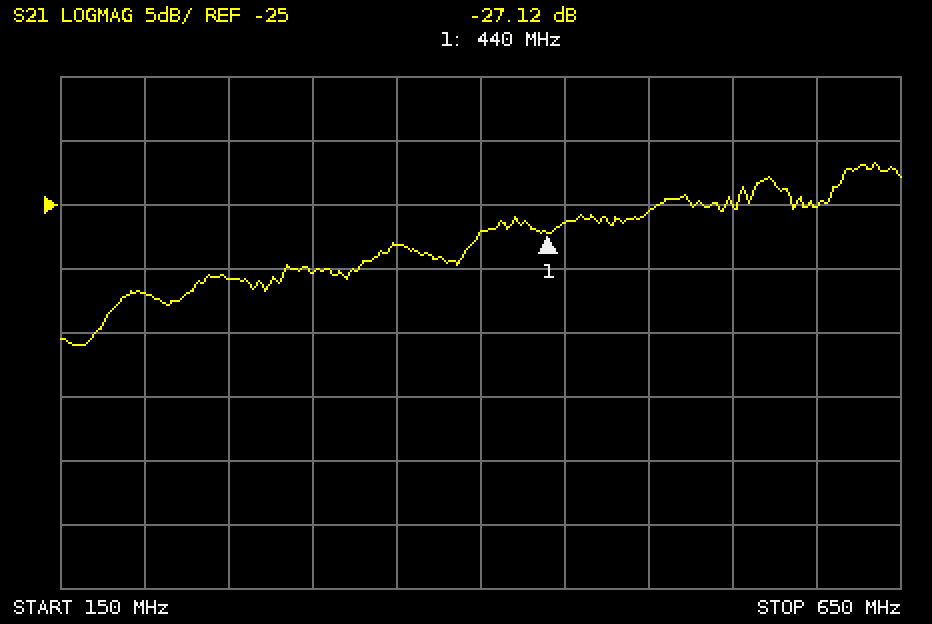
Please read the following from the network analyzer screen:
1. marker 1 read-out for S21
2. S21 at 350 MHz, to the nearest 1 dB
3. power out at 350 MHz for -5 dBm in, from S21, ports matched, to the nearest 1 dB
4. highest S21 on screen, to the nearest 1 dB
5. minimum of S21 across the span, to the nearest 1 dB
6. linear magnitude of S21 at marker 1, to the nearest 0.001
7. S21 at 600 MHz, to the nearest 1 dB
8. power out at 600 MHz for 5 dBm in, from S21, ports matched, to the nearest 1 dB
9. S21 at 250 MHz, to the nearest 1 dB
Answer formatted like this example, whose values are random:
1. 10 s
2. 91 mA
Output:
1. -27.12 dB
2. -28 dB
3. -33 dBm
4. -22 dB
5. -36 dB
6. 0.044
7. -25 dB
8. -20 dBm
9. -31 dB
